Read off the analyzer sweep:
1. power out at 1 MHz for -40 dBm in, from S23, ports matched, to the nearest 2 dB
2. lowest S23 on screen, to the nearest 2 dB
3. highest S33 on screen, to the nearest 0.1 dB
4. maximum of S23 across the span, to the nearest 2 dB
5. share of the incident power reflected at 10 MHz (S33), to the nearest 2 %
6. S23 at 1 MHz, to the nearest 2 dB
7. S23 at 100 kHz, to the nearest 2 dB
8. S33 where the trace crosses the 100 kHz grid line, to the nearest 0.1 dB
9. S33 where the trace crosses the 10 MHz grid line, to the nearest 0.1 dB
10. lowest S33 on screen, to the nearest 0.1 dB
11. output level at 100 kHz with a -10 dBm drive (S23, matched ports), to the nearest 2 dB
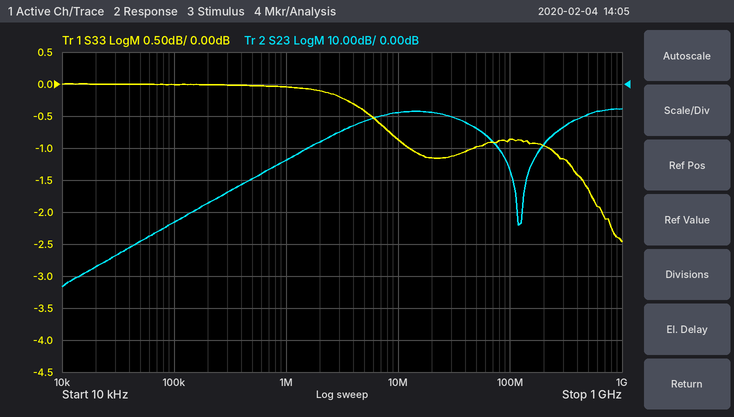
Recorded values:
-64 dBm
-64 dB
0.0 dB
-8 dB
82 %
-24 dB
-44 dB
0.0 dB
-0.9 dB
-2.5 dB
-54 dBm
